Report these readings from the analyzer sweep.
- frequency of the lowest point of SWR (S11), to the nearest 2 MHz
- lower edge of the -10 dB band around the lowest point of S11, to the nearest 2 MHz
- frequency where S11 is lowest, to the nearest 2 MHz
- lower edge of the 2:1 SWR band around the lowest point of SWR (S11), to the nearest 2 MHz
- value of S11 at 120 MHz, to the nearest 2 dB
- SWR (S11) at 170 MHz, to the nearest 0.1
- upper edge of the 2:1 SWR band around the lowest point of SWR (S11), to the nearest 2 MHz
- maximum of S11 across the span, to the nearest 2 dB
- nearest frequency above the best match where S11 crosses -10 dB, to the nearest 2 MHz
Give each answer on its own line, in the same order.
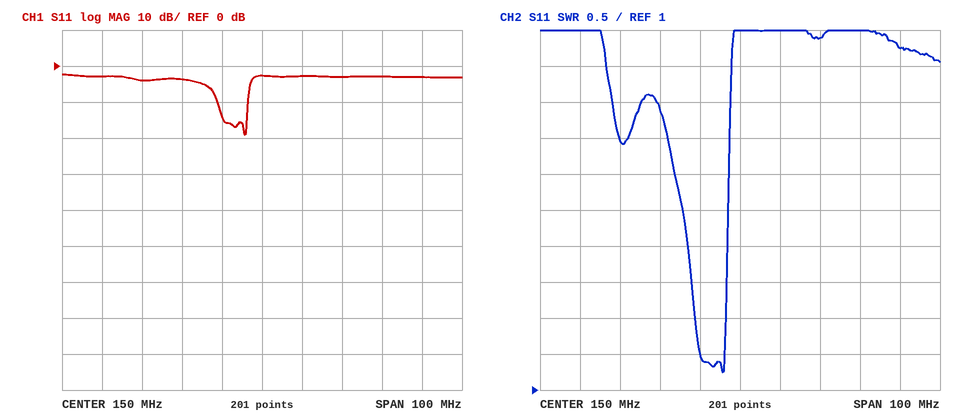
146 MHz
138 MHz
146 MHz
138 MHz
-4 dB
5.9
146 MHz
-2 dB
146 MHz
